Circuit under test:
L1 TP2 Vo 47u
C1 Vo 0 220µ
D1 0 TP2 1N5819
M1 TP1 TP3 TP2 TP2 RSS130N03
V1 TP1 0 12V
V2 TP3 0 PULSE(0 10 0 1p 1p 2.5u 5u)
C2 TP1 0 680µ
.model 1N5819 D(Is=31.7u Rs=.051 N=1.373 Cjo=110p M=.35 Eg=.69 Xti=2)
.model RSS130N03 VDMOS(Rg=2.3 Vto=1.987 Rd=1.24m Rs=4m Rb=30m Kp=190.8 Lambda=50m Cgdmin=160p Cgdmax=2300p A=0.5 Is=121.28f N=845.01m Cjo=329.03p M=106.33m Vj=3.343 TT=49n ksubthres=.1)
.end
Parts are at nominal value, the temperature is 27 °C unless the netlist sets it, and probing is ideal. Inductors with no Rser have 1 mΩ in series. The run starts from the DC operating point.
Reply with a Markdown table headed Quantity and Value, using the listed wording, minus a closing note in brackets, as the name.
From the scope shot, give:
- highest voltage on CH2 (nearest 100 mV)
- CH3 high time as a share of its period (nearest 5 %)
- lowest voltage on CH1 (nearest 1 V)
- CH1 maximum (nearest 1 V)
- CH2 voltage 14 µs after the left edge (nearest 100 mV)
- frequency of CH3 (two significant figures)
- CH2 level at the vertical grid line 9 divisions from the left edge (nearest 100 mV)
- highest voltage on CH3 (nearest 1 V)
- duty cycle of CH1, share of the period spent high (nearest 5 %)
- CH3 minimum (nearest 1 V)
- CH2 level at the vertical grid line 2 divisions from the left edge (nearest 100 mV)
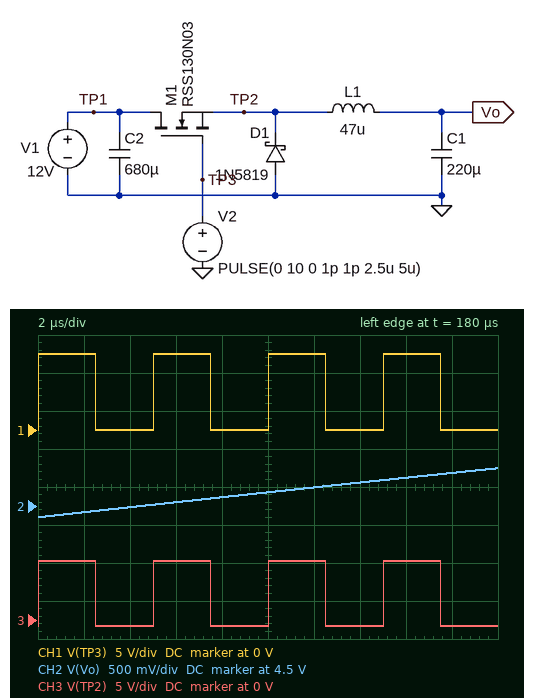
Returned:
| Quantity | Value |
|---|---|
| highest voltage on CH2 | 5.0 V |
| CH3 high time as a share of its period | 50 % |
| lowest voltage on CH1 | 0 V |
| CH1 maximum | 10 V |
| CH2 voltage 14 µs after the left edge | 4.8 V |
| frequency of CH3 | 200 kHz |
| CH2 level at the vertical grid line 9 divisions from the left edge | 4.9 V |
| highest voltage on CH3 | 8 V |
| duty cycle of CH1, share of the period spent high | 50 % |
| CH3 minimum | -1 V |
| CH2 level at the vertical grid line 2 divisions from the left edge | 4.5 V |
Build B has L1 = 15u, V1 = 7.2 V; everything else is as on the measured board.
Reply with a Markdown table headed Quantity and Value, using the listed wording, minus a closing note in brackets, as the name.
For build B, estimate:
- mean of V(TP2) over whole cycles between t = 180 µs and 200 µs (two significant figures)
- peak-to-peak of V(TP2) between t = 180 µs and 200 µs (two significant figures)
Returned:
| Quantity | Value |
|---|---|
| mean of V(TP2) over whole cycles between t = 180 µs and 200 µs | 6.2 V |
| peak-to-peak of V(TP2) between t = 180 µs and 200 µs | 8.2 V |
